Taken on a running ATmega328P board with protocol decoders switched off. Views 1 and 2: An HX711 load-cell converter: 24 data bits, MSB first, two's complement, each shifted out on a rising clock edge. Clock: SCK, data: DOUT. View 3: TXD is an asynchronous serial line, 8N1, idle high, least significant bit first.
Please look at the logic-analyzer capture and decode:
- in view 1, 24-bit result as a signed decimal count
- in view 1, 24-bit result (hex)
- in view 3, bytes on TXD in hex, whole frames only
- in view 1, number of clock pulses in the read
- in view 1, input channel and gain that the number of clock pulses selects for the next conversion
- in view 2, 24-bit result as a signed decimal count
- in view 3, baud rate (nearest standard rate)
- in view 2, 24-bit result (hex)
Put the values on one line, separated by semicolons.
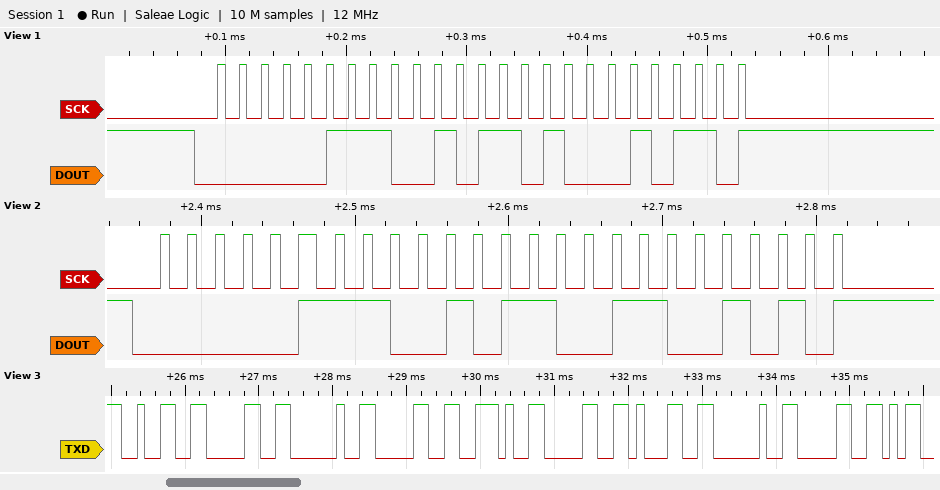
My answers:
470294; 0x072D16; 32 30 20 30 2E 30 31 20 30; 25; channel A, gain 128; 470218; 9600 baud; 0x072CCA
